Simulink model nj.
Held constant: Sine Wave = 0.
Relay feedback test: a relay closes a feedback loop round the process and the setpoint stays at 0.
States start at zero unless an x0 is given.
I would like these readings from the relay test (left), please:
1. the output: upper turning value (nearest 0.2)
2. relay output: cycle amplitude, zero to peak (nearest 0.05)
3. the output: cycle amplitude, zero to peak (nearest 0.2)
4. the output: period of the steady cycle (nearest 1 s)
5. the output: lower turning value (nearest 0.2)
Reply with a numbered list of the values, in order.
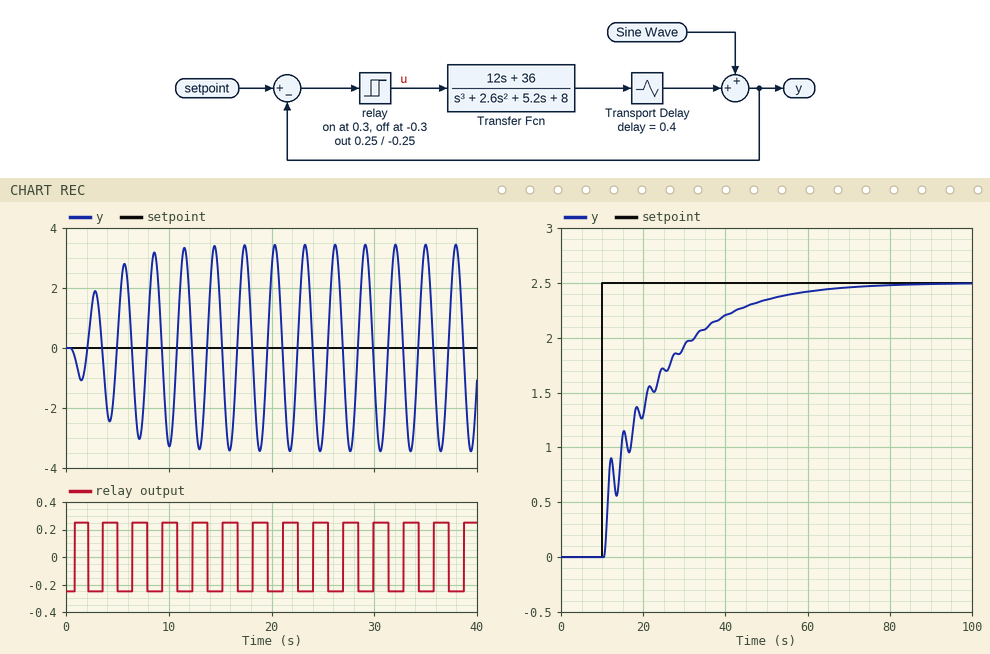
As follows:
1. 3.4
2. 0.25
3. 3.4
4. 3 s
5. -3.4
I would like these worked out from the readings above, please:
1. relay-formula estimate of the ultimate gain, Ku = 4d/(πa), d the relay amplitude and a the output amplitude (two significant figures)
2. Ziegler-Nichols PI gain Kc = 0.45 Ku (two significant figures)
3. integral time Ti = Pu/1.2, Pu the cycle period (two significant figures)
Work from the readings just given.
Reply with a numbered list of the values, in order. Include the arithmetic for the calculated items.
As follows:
1. 4 × 0.25 / (π × 3.4) = 0.094
2. 0.45 × 0.094 = 0.042
3. 3 / 1.2 = 2.5 s
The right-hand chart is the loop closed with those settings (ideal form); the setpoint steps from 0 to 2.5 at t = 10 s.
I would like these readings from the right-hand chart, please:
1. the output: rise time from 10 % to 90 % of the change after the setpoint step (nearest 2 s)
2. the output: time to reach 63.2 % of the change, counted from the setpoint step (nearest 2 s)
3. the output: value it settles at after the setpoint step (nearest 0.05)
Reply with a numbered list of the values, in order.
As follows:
1. 32 s
2. 14 s
3. 2.50
